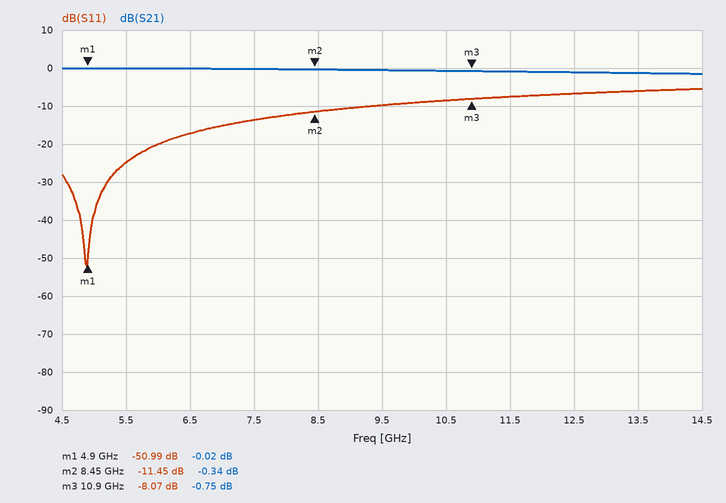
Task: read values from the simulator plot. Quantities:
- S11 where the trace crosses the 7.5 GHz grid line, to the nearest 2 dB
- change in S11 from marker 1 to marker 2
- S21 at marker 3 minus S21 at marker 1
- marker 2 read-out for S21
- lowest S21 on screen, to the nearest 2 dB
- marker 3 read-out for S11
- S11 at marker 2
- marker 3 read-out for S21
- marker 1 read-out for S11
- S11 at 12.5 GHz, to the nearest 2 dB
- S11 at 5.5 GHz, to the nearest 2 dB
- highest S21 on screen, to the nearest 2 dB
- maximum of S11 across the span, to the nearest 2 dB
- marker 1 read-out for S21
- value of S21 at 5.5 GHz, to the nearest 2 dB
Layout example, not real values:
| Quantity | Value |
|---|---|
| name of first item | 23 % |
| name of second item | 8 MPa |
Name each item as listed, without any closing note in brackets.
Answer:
| Quantity | Value |
|---|---|
| S11 where the trace crosses the 7.5 GHz grid line, to the nearest 2 dB | -14 dB |
| change in S11 from marker 1 to marker 2 | 39.54 dB |
| S21 at marker 3 minus S21 at marker 1 | -0.73 dB |
| marker 2 read-out for S21 | -0.34 dB |
| lowest S21 on screen, to the nearest 2 dB | -2 dB |
| marker 3 read-out for S11 | -8.07 dB |
| S11 at marker 2 | -11.45 dB |
| marker 3 read-out for S21 | -0.75 dB |
| marker 1 read-out for S11 | -50.99 dB |
| S11 at 12.5 GHz, to the nearest 2 dB | -6 dB |
| S11 at 5.5 GHz, to the nearest 2 dB | -24 dB |
| highest S21 on screen, to the nearest 2 dB | 0 dB |
| maximum of S11 across the span, to the nearest 2 dB | -6 dB |
| marker 1 read-out for S21 | -0.02 dB |
| value of S21 at 5.5 GHz, to the nearest 2 dB | 0 dB |
